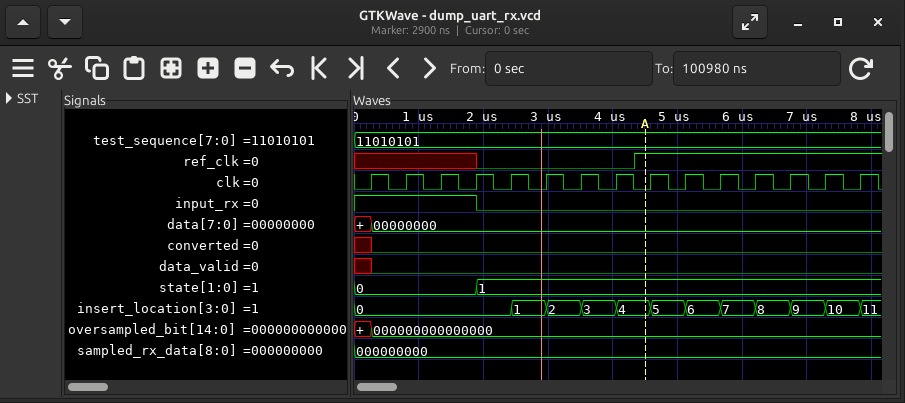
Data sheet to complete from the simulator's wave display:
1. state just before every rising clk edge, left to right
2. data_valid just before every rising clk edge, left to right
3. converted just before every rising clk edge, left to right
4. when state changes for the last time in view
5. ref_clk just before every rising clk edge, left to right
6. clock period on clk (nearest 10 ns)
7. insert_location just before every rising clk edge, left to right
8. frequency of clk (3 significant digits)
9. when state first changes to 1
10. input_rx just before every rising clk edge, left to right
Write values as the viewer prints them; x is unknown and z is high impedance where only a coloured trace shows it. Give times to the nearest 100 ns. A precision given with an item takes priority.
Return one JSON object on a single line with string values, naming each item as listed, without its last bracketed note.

{"state just before every rising clk edge, left to right": "0, 0, 0, 0, 1, 1, 1, 1, 1, 1, 1, 1, 1, 1, 1", "data_valid just before every rising clk edge, left to right": "x 0 0 0 0 0 0 0 0 0 0 0 0 0 0", "converted just before every rising clk edge, left to right": "x 0 0 0 0 0 0 0 0 0 0 0 0 0 0", "when state changes for the last time in view": "1900 ns", "ref_clk just before every rising clk edge, left to right": "x x x x 0 0 0 0 1 1 1 1 1 1 1", "clock period on clk": "540 ns", "insert_location just before every rising clk edge, left to right": "0, 0, 0, 0, 0, 1, 2, 3, 4, 5, 6, 7, 8, 9, 10", "frequency of clk": "1.85 MHz", "when state first changes to 1": "1900 ns", "input_rx just before every rising clk edge, left to right": "1 1 1 1 0 0 0 0 0 0 0 0 0 0 0"}
